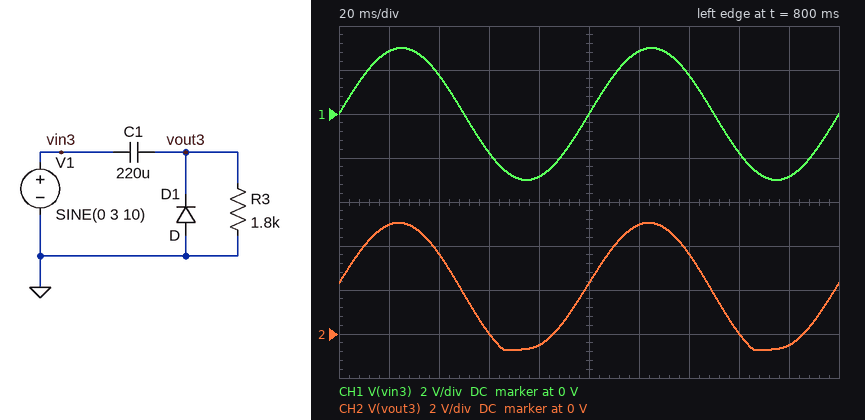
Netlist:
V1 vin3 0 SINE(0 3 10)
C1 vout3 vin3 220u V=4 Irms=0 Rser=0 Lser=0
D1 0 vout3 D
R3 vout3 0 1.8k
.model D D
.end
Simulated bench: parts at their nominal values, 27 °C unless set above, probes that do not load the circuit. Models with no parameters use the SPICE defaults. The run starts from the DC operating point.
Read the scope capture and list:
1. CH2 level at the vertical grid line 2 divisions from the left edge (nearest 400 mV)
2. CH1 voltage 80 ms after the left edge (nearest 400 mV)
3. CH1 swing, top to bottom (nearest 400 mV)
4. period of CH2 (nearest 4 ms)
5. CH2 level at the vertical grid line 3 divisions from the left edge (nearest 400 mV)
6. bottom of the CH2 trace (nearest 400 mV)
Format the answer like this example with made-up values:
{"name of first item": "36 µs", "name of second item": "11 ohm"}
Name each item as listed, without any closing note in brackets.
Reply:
{"CH2 level at the vertical grid line 2 divisions from the left edge": "3.6 V", "CH1 voltage 80 ms after the left edge": "-2.8 V", "CH1 swing, top to bottom": "6.0 V", "period of CH2": "100 ms", "CH2 level at the vertical grid line 3 divisions from the left edge": "0 V", "bottom of the CH2 trace": "-800 mV"}
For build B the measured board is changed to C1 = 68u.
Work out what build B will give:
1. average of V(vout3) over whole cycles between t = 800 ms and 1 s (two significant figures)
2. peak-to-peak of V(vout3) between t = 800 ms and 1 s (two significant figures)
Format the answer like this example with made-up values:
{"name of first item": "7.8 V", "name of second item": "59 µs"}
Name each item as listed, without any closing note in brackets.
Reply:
{"average of V(vout3) over whole cycles between t = 800 ms and 1 s": "1.7 V", "peak-to-peak of V(vout3) between t = 800 ms and 1 s": "5.3 V"}
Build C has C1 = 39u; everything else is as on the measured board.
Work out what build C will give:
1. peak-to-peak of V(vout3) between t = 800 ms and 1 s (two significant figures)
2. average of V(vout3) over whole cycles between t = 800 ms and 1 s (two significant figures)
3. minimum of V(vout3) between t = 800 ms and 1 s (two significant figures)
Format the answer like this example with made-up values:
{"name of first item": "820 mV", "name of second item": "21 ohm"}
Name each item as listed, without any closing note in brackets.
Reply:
{"peak-to-peak of V(vout3) between t = 800 ms and 1 s": "4.8 V", "average of V(vout3) over whole cycles between t = 800 ms and 1 s": "1.4 V", "minimum of V(vout3) between t = 800 ms and 1 s": "-700 mV"}
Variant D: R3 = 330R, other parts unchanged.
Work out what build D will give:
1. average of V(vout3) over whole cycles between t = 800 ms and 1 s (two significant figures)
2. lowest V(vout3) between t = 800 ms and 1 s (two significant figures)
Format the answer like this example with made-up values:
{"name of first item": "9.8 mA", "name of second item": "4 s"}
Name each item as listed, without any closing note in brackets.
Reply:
{"average of V(vout3) over whole cycles between t = 800 ms and 1 s": "1.4 V", "lowest V(vout3) between t = 800 ms and 1 s": "-750 mV"}
